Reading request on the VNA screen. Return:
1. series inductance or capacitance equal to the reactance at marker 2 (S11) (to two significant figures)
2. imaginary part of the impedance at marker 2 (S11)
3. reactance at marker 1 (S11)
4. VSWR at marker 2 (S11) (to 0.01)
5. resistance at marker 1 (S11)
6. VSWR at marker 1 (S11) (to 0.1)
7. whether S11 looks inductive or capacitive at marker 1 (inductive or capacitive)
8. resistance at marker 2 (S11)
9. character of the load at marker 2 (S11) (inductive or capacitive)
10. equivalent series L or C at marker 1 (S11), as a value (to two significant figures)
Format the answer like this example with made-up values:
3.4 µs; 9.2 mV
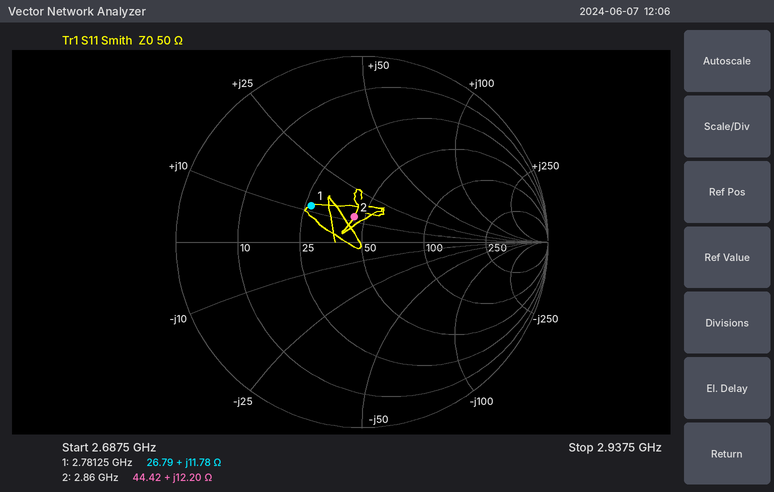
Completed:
680 pH; +12.20 Ω; +11.78 Ω; 1.33; 26.79 Ω; 2.0; inductive; 44.42 Ω; inductive; 670 pH
